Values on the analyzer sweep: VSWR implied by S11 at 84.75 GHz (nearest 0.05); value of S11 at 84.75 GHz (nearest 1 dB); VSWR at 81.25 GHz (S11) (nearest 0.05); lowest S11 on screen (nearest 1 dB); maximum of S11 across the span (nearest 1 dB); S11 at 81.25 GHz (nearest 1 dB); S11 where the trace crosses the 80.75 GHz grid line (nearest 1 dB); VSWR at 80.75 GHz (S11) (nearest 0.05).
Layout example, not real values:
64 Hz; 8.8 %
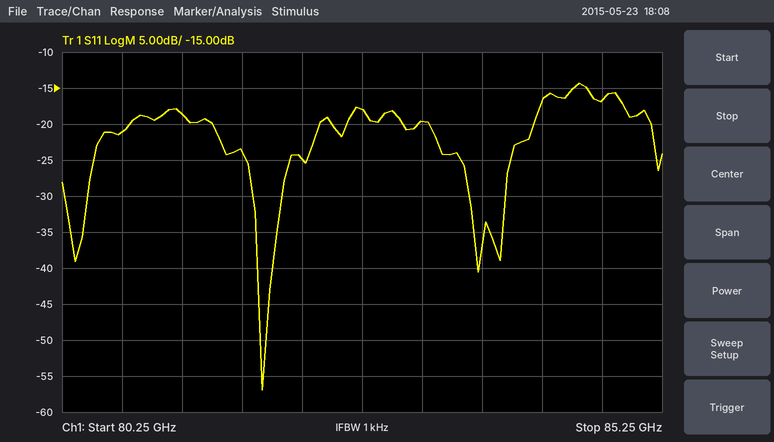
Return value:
1.35; -17 dB; 1.25; -57 dB; -14 dB; -19 dB; -21 dB; 1.20
